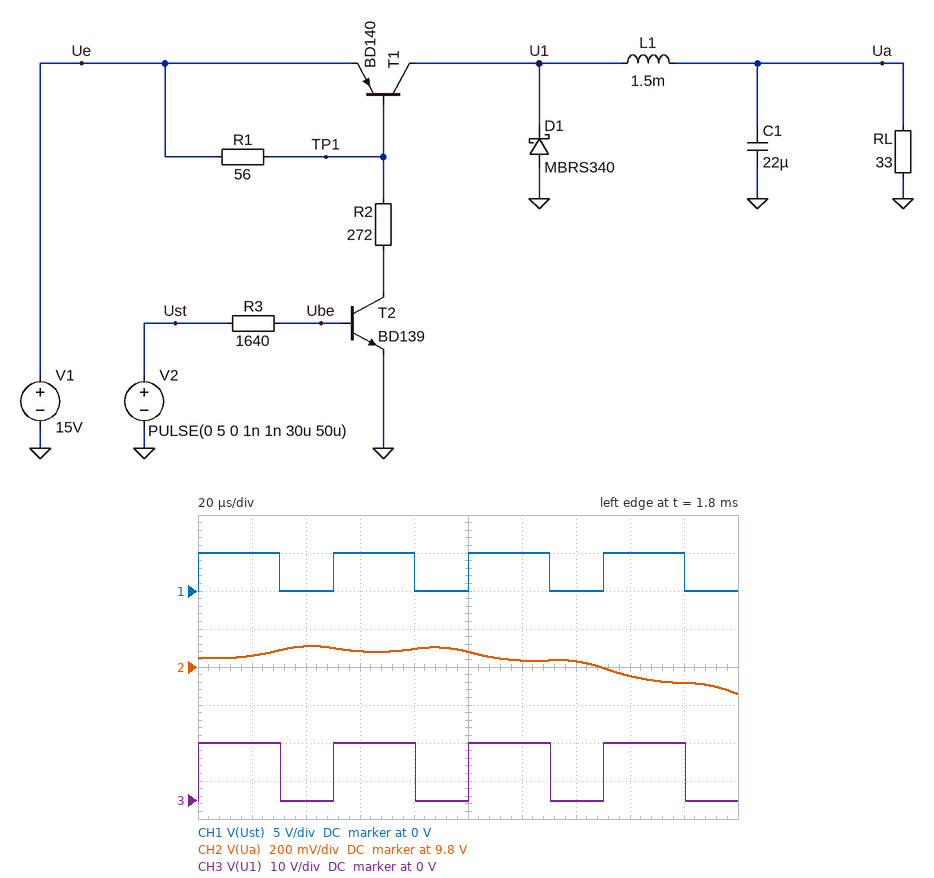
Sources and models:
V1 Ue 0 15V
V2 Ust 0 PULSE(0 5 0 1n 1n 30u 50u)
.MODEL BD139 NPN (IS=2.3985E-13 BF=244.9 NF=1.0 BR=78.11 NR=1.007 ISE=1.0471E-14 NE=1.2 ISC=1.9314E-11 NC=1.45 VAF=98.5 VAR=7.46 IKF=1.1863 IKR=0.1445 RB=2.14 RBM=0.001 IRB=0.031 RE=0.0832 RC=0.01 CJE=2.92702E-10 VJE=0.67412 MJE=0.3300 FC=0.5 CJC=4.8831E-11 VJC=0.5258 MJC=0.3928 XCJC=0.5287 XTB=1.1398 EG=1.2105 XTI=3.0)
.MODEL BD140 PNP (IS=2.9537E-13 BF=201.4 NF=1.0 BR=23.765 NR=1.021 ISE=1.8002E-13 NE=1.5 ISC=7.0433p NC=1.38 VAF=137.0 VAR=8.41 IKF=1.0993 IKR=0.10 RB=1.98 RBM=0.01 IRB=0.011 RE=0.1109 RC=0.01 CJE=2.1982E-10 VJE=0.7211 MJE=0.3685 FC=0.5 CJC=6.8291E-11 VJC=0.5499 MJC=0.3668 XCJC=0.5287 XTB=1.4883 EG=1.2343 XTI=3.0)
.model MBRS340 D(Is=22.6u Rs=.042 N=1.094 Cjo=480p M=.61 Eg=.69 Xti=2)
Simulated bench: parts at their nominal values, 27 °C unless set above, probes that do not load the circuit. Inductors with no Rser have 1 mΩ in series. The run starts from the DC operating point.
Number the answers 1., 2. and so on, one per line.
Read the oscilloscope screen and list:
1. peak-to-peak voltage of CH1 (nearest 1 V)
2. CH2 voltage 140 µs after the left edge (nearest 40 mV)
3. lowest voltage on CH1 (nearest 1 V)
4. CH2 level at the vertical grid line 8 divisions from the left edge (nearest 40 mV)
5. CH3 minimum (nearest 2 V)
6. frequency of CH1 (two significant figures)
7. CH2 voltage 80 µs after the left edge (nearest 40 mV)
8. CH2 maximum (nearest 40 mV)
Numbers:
1. 5 V
2. 9.84 V
3. 0 V
4. 9.76 V
5. 0 V
6. 20 kHz
7. 9.88 V
8. 9.92 V
